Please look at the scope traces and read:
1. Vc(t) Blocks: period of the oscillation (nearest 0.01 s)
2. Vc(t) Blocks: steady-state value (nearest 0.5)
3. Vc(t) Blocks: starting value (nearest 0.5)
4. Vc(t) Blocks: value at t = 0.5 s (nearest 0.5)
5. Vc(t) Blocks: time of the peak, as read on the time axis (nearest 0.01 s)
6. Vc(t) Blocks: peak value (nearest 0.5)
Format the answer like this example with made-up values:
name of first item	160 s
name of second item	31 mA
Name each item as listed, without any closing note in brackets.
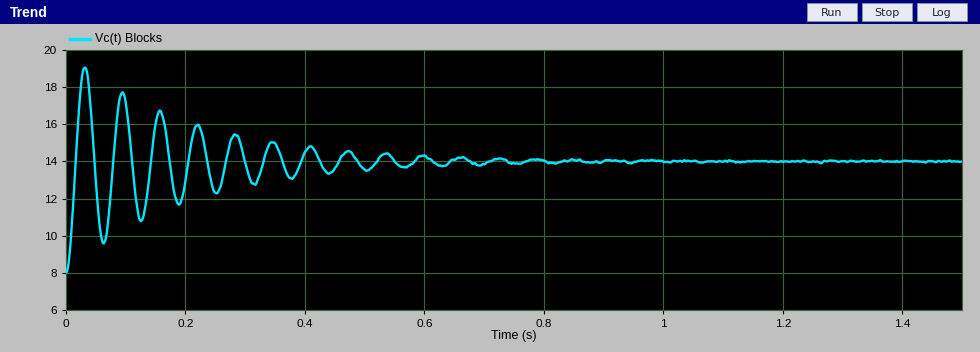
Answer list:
Vc(t) Blocks: period of the oscillation	0.06 s
Vc(t) Blocks: steady-state value	14.0
Vc(t) Blocks: starting value	8.0
Vc(t) Blocks: value at t = 0.5 s	13.5
Vc(t) Blocks: time of the peak, as read on the time axis	0.03 s
Vc(t) Blocks: peak value	19.0
